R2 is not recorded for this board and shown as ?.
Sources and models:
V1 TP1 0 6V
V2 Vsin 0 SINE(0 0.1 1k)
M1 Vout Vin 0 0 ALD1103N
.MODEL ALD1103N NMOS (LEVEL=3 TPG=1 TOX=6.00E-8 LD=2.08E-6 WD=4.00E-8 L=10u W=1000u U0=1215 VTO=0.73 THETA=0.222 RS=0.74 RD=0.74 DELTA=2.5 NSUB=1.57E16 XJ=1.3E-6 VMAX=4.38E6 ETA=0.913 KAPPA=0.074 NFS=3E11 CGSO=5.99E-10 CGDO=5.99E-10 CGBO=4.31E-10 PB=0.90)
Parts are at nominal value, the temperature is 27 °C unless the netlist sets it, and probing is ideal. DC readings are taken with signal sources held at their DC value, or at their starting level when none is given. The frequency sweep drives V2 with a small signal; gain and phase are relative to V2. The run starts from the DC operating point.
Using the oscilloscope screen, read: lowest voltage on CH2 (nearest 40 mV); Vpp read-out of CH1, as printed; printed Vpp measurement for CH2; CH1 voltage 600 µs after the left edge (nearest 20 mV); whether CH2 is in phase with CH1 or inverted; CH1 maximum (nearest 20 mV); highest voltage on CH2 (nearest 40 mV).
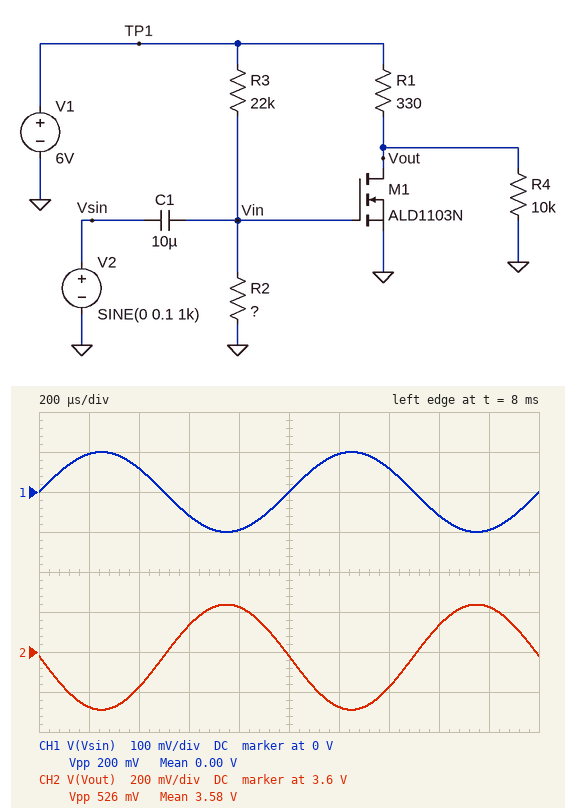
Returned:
3.32 V
200 mV
526 mV
-60 mV
inverted
100 mV
3.84 V
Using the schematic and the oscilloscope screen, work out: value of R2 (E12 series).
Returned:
12 kΩ
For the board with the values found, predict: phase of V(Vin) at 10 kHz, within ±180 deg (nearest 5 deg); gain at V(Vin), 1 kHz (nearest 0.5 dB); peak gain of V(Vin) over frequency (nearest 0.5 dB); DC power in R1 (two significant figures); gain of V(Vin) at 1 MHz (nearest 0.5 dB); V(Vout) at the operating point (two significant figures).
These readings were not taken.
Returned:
0 deg
0 dB
0 dB
18 mW
0 dB
3.6 V
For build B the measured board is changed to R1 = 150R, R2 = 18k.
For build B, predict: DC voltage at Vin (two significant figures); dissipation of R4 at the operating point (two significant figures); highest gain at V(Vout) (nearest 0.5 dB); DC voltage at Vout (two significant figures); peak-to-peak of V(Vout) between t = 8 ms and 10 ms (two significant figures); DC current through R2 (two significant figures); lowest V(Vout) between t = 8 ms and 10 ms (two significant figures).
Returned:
2.7 V
1.7 mW
3.5 dB
4.1 V
300 mV
150 µA
3.9 V
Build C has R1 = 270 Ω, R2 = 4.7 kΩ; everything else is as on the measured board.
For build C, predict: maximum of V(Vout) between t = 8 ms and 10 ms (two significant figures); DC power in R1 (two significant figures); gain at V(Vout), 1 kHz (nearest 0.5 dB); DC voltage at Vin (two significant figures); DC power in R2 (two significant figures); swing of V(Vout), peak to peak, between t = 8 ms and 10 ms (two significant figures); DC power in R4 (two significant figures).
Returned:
5.7 V
410 µW
-1.5 dB
1.1 V
240 µW
160 mV
3.2 mW
